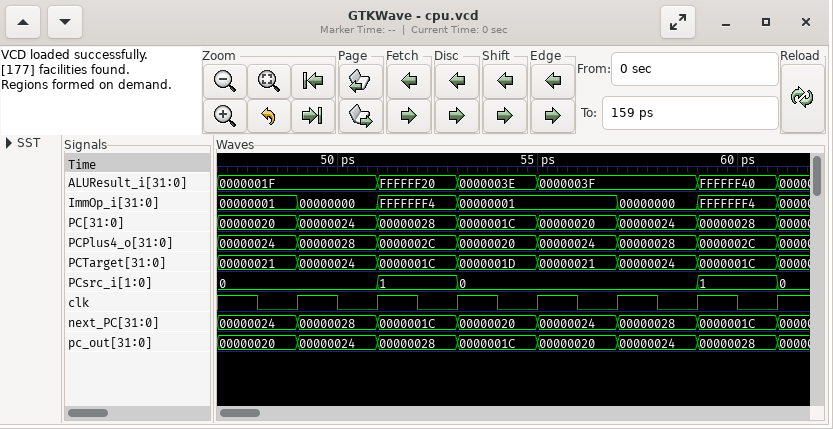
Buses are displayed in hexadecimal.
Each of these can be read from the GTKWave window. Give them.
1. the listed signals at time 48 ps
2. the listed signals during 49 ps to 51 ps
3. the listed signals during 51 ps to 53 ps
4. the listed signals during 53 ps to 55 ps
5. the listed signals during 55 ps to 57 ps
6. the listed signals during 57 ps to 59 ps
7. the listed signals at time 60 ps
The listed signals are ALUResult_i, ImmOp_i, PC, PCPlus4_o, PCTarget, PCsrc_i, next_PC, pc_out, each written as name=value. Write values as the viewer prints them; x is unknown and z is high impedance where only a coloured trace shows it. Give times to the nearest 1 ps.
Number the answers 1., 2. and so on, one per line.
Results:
1. ALUResult_i=0000001F, ImmOp_i=00000001, PC=00000020, PCPlus4_o=00000024, PCTarget=00000021, PCsrc_i=0, next_PC=00000024, pc_out=00000020
2. ALUResult_i=0000001F, ImmOp_i=00000000, PC=00000024, PCPlus4_o=00000028, PCTarget=00000024, PCsrc_i=0, next_PC=00000028, pc_out=00000024
3. ALUResult_i=FFFFFF20, ImmOp_i=FFFFFFF4, PC=00000028, PCPlus4_o=0000002C, PCTarget=0000001C, PCsrc_i=1, next_PC=0000001C, pc_out=00000028
4. ALUResult_i=0000003E, ImmOp_i=00000001, PC=0000001C, PCPlus4_o=00000020, PCTarget=0000001D, PCsrc_i=0, next_PC=00000020, pc_out=0000001C
5. ALUResult_i=0000003F, ImmOp_i=00000001, PC=00000020, PCPlus4_o=00000024, PCTarget=00000021, PCsrc_i=0, next_PC=00000024, pc_out=00000020
6. ALUResult_i=0000003F, ImmOp_i=00000000, PC=00000024, PCPlus4_o=00000028, PCTarget=00000024, PCsrc_i=0, next_PC=00000028, pc_out=00000024
7. ALUResult_i=FFFFFF40, ImmOp_i=FFFFFFF4, PC=00000028, PCPlus4_o=0000002C, PCTarget=0000001C, PCsrc_i=1, next_PC=0000001C, pc_out=00000028
